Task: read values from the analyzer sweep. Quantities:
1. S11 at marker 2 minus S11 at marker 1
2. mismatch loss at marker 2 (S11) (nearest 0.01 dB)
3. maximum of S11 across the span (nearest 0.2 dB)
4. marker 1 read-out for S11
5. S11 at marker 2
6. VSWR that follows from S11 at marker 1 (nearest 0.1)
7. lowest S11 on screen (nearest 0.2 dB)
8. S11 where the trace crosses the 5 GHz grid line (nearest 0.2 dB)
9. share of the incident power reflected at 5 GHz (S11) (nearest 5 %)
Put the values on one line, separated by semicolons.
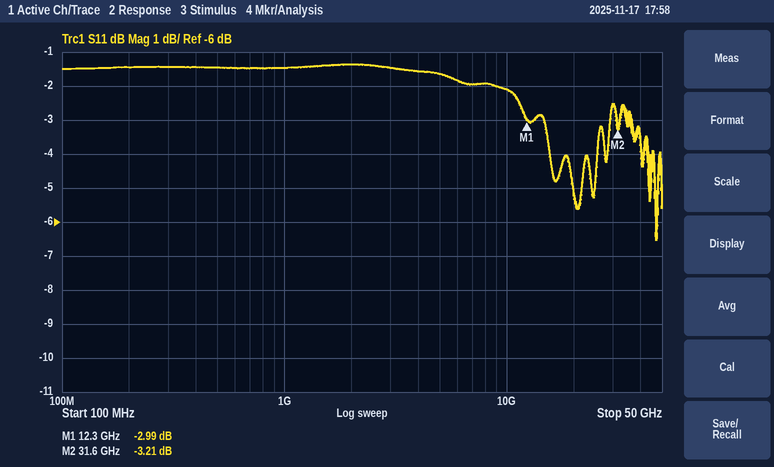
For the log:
-0.22 dB; 2.82 dB; -1.4 dB; -2.99 dB; -3.21 dB; 5.9; -6.6 dB; -1.6 dB; 70 %
